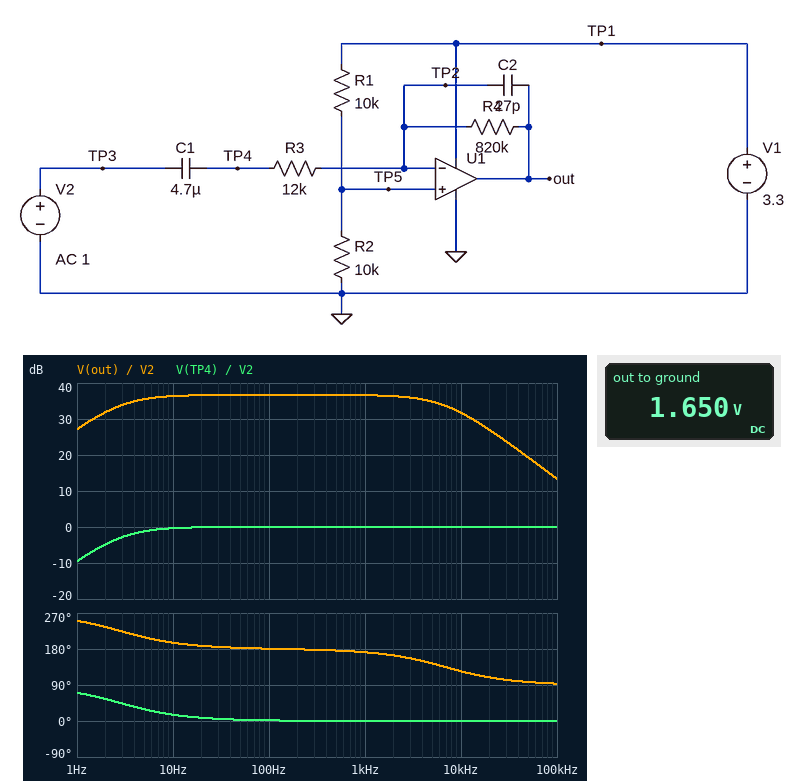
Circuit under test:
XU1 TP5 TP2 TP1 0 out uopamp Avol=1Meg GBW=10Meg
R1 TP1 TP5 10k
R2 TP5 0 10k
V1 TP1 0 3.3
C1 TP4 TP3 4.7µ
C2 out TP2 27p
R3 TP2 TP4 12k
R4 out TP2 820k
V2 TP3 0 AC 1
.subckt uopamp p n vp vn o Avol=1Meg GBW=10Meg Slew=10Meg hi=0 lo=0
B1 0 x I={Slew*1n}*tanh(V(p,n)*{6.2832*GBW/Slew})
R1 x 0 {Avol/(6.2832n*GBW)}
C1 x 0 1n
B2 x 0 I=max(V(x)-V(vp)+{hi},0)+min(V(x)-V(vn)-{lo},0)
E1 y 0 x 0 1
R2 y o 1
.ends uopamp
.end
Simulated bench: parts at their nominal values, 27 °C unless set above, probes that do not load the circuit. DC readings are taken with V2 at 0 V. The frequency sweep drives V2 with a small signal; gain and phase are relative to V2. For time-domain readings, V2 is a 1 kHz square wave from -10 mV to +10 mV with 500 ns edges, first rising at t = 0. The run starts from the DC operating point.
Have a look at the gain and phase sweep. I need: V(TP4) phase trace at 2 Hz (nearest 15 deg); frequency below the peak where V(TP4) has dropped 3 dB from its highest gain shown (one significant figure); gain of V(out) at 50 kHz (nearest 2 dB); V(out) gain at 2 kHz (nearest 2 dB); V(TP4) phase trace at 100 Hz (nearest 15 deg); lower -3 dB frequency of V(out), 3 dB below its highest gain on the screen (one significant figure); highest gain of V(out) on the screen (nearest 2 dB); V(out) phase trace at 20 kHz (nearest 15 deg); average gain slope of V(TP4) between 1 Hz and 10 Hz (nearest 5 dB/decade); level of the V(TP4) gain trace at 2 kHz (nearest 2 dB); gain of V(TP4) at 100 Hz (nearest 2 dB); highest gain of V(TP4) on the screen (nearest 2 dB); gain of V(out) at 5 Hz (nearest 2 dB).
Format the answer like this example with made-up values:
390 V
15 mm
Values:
60 deg
3 Hz
20 dB
36 dB
0 deg
3 Hz
36 dB
105 deg
10 dB/decade
0 dB
0 dB
0 dB
36 dB
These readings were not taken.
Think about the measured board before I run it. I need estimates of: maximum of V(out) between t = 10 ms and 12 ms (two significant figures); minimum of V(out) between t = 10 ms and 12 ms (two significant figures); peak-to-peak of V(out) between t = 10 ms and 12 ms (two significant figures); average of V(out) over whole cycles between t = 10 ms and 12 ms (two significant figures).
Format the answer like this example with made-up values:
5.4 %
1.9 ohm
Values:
1.8 V
400 mV
1.4 V
1.1 V
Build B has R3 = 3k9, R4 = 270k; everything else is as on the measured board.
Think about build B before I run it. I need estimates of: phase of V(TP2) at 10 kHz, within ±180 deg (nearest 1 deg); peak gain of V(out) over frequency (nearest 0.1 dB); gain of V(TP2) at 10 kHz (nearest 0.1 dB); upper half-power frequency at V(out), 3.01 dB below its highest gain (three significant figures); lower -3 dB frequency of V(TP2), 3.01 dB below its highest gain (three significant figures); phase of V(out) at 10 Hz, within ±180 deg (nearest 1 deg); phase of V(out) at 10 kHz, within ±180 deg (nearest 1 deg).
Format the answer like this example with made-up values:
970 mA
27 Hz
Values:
62 deg
36.8 dB
-24.3 dB
19.0 kHz
18.9 kHz
-139 deg
152 deg
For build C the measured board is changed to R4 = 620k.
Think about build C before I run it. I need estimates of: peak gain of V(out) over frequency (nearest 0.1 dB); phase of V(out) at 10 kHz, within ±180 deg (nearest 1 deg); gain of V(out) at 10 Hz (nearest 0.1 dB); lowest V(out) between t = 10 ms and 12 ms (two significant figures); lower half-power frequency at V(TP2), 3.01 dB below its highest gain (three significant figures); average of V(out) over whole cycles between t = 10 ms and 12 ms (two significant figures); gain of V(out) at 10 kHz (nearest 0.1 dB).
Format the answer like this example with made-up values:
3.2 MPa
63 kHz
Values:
34.3 dB
132 deg
33.9 dB
700 mV
9.05 kHz
1.2 V
30.8 dB
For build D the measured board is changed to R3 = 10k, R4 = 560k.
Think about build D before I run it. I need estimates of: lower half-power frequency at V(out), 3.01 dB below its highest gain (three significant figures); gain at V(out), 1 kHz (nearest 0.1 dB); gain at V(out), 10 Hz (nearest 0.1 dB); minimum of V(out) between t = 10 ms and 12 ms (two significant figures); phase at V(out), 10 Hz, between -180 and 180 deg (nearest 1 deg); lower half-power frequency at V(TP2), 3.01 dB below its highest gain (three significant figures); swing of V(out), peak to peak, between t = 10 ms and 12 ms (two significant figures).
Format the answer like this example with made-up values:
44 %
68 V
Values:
3.38 Hz
34.9 dB
34.5 dB
640 mV
-161 deg
9.92 kHz
1.1 V
